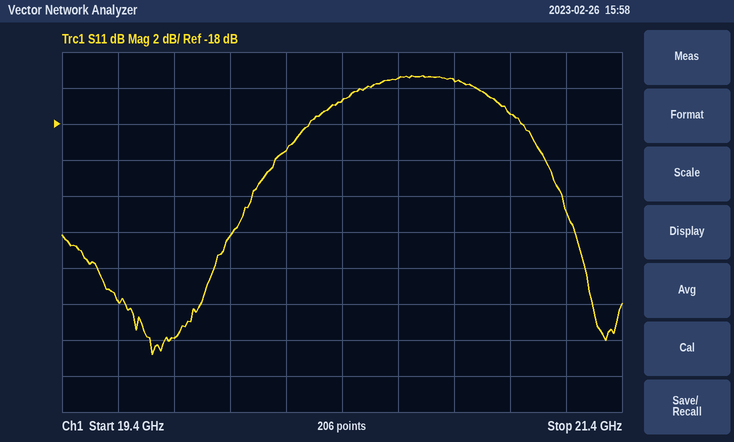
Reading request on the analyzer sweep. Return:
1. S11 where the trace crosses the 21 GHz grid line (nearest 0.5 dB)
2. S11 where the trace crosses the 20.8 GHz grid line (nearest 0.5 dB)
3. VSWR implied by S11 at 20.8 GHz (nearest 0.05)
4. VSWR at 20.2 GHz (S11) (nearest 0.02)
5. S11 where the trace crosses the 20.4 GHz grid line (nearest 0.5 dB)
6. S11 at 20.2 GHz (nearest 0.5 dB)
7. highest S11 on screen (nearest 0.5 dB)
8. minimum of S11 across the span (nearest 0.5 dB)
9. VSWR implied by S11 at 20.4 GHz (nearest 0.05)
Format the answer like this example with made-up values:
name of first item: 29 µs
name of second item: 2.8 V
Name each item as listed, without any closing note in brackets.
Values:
S11 where the trace crosses the 21 GHz grid line: -17.5 dB
S11 where the trace crosses the 20.8 GHz grid line: -15.5 dB
VSWR implied by S11 at 20.8 GHz: 1.40
VSWR at 20.2 GHz (S11): 1.24
S11 where the trace crosses the 20.4 GHz grid line: -16.5 dB
S11 at 20.2 GHz: -19.5 dB
highest S11 on screen: -15.5 dB
minimum of S11 across the span: -31.0 dB
VSWR implied by S11 at 20.4 GHz: 1.35
